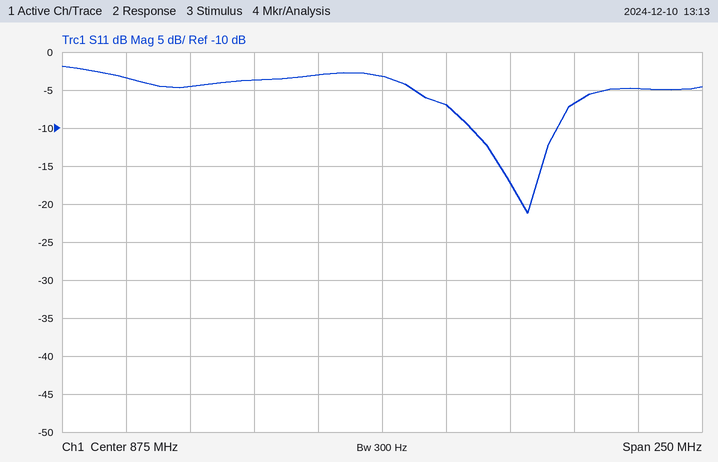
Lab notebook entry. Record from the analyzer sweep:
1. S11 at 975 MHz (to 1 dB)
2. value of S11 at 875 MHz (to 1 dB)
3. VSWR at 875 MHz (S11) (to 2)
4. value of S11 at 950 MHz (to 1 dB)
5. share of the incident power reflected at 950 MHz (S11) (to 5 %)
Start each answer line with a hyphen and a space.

- -5 dB
- -3 dB
- 6
- -7 dB
- 20 %
